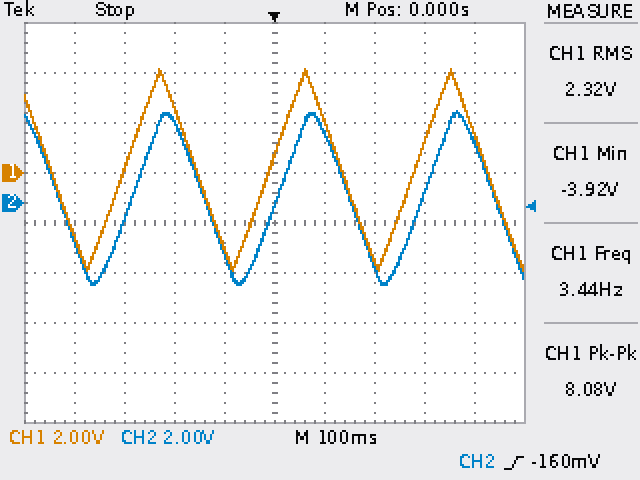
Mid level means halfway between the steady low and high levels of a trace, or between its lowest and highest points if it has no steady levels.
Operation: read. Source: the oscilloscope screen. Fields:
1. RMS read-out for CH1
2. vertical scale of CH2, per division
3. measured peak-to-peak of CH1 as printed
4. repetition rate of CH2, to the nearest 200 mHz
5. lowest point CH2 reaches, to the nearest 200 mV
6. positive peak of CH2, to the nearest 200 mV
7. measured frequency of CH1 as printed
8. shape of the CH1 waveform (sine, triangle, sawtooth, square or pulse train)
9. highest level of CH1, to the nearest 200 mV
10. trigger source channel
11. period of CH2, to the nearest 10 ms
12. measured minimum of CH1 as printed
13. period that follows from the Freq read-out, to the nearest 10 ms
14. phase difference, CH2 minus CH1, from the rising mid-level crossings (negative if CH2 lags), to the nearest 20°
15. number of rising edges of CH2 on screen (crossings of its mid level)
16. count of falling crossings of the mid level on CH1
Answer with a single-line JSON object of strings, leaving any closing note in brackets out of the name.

{"RMS read-out for CH1": "2.32 V", "vertical scale of CH2, per division": "2 V", "measured peak-to-peak of CH1 as printed": "8.08 V", "repetition rate of CH2, to the nearest 200 mHz": "3.4 Hz", "lowest point CH2 reaches, to the nearest 200 mV": "-3.2 V", "positive peak of CH2, to the nearest 200 mV": "3.6 V", "measured frequency of CH1 as printed": "3.44 Hz", "shape of the CH1 waveform": "triangle", "highest level of CH1, to the nearest 200 mV": "4.2 V", "trigger source channel": "CH2", "period of CH2, to the nearest 10 ms": "290 ms", "measured minimum of CH1 as printed": "-3.92 V", "period that follows from the Freq read-out, to the nearest 10 ms": "290 ms", "phase difference, CH2 minus CH1, from the rising mid-level crossings (negative if CH2 lags), to the nearest 20°": "-20°", "number of rising edges of CH2 on screen": "3", "count of falling crossings of the mid level on CH1": "4"}
